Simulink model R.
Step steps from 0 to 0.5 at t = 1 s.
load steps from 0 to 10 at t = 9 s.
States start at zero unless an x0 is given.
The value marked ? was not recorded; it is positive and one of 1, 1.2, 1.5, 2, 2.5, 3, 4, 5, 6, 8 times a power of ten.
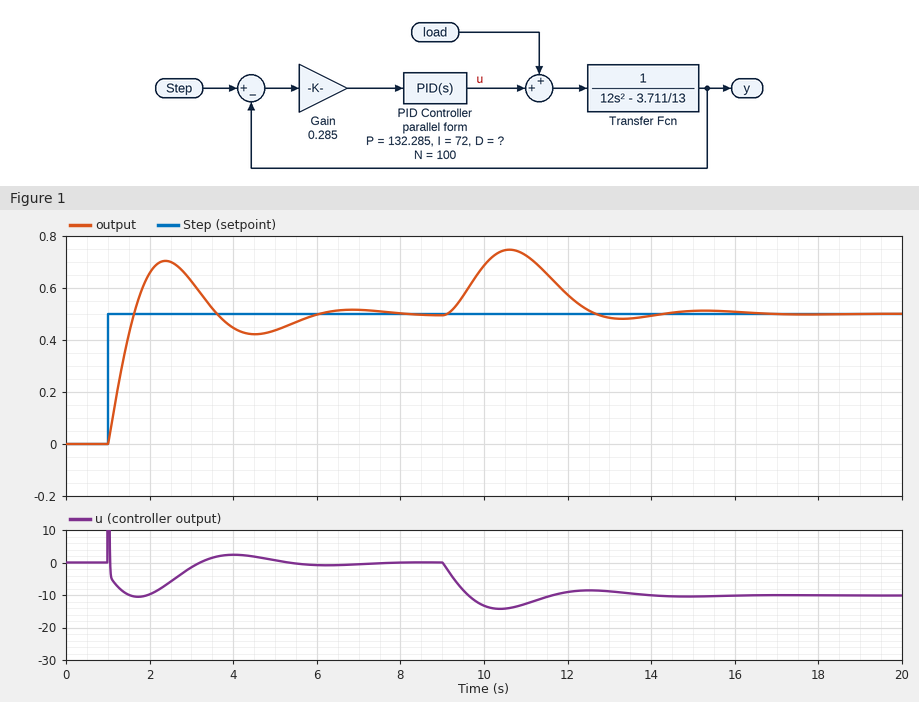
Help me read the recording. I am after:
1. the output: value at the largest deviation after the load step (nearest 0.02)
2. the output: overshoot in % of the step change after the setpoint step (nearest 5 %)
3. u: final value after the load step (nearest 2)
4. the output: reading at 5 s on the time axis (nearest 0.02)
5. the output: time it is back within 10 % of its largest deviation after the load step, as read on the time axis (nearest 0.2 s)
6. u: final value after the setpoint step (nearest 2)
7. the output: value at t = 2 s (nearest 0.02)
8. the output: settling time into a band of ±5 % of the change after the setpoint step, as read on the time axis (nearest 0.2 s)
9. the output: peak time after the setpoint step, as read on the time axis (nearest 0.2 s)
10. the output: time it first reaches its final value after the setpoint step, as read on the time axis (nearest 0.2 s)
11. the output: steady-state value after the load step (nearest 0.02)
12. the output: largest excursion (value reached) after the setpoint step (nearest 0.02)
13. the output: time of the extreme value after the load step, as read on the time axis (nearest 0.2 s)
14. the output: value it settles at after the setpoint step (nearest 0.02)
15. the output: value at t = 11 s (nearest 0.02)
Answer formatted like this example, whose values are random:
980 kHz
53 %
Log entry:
0.74
40 %
-10
0.44
12.4 s
0
0.66
5.6 s
2.4 s
1.6 s
0.50
0.70
10.6 s
0.50
0.72
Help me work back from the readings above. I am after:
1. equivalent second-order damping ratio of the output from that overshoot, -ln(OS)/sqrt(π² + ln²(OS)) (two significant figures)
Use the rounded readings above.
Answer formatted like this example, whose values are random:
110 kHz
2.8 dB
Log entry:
0.28
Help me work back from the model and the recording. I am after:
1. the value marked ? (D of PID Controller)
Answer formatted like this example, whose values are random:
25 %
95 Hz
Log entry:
80
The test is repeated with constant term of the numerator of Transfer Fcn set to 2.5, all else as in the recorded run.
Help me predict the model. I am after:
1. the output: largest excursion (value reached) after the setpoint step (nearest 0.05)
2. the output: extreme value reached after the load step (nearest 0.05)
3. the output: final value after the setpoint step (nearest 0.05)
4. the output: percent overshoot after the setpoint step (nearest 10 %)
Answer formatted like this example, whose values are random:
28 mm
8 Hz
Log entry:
0.60
0.70
0.50
20 %
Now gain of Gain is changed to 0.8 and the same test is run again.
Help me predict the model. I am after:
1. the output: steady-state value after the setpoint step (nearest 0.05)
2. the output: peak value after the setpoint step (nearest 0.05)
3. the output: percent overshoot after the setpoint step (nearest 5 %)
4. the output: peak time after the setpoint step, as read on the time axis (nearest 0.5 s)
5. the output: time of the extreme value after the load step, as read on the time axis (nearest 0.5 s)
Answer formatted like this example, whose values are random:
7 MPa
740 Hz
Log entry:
0.50
0.60
20 %
1.5 s
10.0 s
